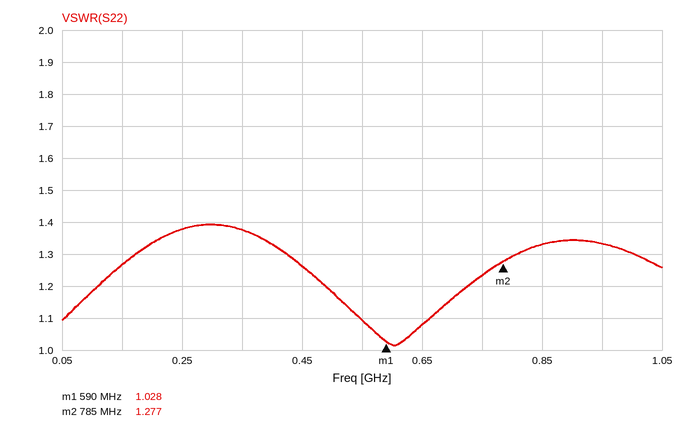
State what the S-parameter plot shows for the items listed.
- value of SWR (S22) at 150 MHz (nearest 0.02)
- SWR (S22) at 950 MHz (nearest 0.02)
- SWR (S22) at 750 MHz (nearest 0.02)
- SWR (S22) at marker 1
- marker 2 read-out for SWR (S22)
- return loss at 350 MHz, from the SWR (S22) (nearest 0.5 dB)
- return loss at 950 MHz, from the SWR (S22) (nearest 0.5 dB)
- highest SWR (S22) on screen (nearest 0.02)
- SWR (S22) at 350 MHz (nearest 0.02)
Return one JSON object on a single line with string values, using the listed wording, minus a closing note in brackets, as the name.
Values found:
{"value of SWR (S22) at 150 MHz": "1.26", "SWR (S22) at 950 MHz": "1.34", "SWR (S22) at 750 MHz": "1.24", "SWR (S22) at marker 1": "1.028", "marker 2 read-out for SWR": "1.277", "return loss at 350 MHz, from the SWR (S22)": "16.0 dB", "return loss at 950 MHz, from the SWR (S22)": "17.0 dB", "highest SWR (S22) on screen": "1.40", "SWR (S22) at 350 MHz": "1.38"}
